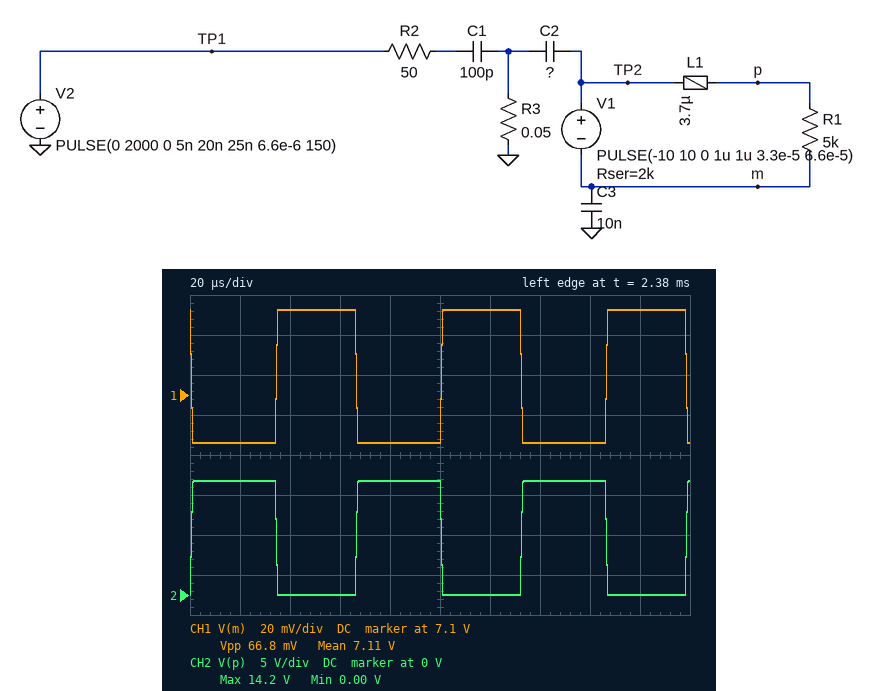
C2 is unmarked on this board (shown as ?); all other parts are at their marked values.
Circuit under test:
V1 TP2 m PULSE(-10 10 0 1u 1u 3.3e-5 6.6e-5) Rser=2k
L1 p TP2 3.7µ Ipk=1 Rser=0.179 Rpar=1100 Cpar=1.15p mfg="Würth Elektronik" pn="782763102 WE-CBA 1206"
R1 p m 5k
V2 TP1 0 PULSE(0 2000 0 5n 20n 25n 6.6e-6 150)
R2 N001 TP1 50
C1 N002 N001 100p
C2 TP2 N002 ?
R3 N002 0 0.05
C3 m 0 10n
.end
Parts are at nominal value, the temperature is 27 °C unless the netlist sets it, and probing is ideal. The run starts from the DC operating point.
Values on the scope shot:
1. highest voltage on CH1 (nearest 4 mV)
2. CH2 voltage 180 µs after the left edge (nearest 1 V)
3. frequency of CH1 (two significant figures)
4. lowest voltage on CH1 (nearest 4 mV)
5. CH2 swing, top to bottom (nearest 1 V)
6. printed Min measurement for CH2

7.144 V
0 V
15 kHz
7.076 V
14 V
0.00 V
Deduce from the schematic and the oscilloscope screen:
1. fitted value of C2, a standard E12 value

47 pF
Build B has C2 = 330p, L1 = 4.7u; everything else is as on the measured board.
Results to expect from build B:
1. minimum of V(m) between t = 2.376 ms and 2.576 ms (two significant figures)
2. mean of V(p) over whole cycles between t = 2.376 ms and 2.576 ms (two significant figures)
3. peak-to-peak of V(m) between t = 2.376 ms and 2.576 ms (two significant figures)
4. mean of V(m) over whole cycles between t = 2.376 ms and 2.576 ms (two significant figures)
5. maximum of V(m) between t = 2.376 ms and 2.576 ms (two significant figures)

6.7 V
7.1 V
460 mV
6.9 V
7.1 V
